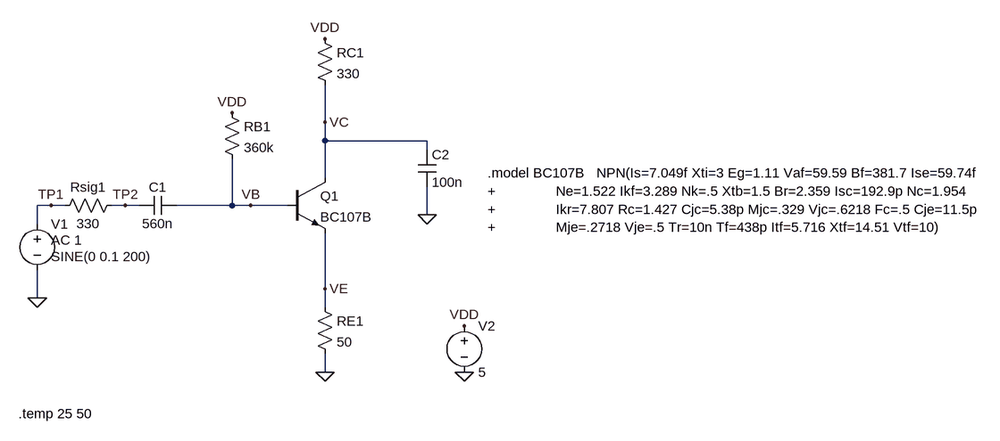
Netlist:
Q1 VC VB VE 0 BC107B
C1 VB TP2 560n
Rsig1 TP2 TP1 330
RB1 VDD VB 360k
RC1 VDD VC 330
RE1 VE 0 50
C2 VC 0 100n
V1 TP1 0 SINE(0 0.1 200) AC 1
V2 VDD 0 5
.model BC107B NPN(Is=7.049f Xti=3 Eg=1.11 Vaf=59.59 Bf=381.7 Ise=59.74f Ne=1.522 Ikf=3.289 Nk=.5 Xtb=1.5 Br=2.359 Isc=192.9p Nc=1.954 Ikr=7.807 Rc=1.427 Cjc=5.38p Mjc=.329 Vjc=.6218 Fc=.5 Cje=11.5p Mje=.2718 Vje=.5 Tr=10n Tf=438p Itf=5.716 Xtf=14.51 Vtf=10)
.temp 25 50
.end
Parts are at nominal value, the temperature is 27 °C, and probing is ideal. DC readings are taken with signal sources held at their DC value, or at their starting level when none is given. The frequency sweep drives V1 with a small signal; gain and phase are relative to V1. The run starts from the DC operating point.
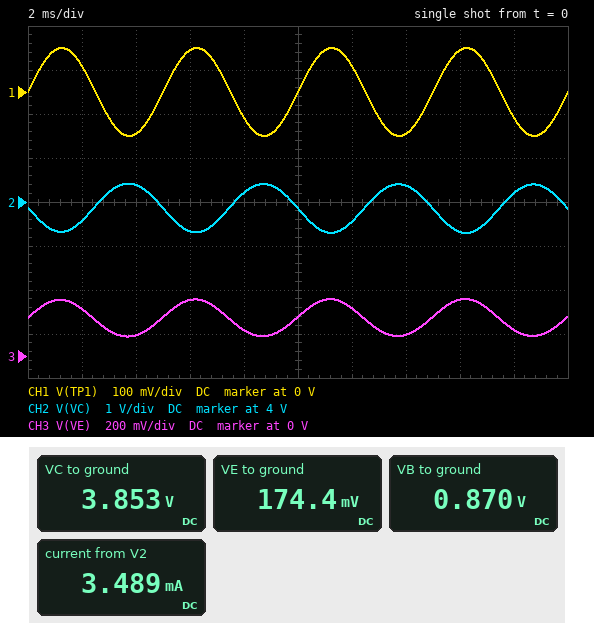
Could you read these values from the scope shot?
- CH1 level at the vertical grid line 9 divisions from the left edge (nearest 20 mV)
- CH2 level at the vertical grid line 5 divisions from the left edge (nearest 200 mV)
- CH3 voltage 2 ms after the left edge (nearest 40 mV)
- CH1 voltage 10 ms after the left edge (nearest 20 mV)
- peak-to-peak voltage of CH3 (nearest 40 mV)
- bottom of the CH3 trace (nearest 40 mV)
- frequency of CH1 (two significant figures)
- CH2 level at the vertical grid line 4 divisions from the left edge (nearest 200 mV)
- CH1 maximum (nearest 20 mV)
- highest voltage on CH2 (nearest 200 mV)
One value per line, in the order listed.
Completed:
-60 mV
3.8 V
200 mV
0 V
160 mV
80 mV
200 Hz
4.2 V
100 mV
4.4 V
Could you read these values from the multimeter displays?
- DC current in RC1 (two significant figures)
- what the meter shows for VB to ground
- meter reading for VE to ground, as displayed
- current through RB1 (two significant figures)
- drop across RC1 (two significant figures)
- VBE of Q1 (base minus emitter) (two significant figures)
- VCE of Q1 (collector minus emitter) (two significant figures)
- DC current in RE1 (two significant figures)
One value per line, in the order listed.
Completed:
3.5 mA
0.870 V
174.4 mV
11 µA
1.1 V
700 mV
3.7 V
3.5 mA
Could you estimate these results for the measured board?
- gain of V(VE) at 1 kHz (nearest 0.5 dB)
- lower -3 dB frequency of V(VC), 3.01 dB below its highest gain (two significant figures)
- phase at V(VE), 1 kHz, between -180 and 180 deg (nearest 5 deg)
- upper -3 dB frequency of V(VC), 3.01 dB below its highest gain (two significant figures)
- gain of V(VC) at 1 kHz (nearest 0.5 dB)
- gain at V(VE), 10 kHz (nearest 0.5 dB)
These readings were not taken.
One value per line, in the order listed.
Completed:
-1.5 dB
16 Hz
0 deg
4.9 kHz
15.0 dB
-1.5 dB
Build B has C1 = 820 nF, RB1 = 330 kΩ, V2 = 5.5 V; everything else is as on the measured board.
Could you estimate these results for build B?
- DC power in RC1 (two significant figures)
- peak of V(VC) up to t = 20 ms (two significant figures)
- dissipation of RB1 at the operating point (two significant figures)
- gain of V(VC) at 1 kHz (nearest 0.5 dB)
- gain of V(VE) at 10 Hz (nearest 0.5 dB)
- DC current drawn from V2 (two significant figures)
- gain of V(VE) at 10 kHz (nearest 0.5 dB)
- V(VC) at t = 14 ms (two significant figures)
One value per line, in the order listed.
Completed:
6.1 mW
4.7 V
64 µW
15.0 dB
-4.5 dB
4.3 mA
-1.0 dB
4.6 V
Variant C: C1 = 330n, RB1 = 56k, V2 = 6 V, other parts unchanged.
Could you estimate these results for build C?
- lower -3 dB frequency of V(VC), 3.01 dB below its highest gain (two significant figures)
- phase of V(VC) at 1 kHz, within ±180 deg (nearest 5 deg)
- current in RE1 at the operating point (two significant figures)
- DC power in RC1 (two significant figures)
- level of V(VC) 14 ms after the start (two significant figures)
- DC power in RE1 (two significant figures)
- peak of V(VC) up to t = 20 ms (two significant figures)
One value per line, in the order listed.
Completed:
840 Hz
-140 deg
15 mA
77 mW
950 mV
12 mW
1.1 V
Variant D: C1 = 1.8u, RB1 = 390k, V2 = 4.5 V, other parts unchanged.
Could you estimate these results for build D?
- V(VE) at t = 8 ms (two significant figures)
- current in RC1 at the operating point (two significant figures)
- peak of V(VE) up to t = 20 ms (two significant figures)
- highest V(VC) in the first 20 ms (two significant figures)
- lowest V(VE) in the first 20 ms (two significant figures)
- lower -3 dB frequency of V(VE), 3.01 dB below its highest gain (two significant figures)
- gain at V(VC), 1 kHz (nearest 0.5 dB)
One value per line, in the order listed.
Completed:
90 mV
2.8 mA
220 mV
4.1 V
61 mV
4.8 Hz
14.5 dB
